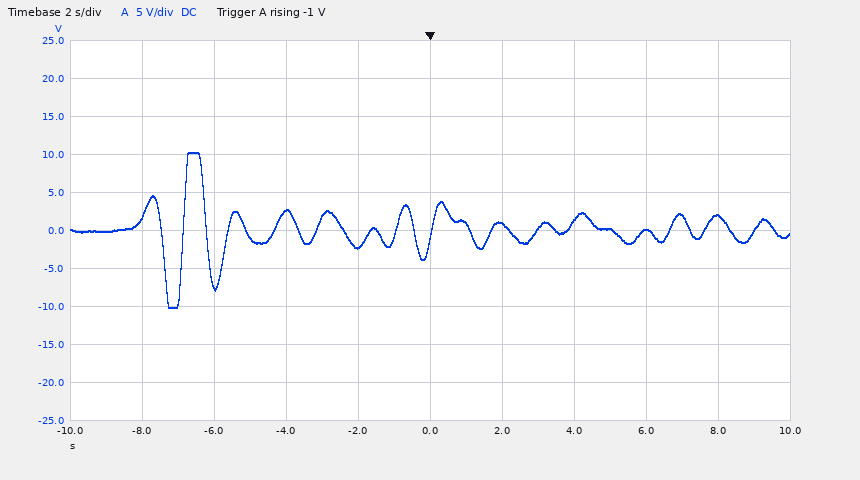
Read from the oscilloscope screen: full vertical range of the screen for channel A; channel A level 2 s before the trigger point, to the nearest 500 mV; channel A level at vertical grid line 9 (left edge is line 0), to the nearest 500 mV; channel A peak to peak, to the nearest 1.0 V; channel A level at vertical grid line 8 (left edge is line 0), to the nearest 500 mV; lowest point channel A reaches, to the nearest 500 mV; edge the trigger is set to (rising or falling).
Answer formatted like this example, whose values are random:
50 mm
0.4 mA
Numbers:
50 V
-2.0 V
2.0 V
20.0 V
0.0 V
-10.0 V
rising
